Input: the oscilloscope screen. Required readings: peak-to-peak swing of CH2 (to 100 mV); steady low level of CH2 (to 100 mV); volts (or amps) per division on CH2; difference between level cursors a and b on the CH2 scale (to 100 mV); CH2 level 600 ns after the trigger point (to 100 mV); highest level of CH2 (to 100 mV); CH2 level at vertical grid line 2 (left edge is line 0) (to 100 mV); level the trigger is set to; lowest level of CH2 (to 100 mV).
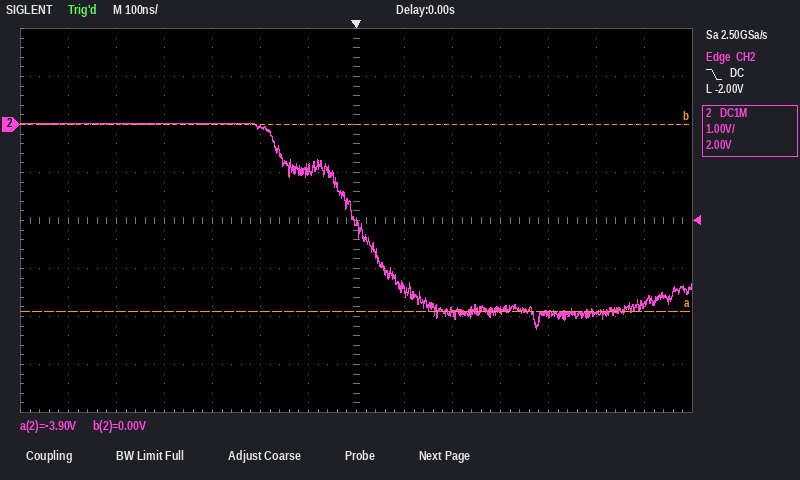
4.3 V
-3.9 V
1 V
3.9 V
-3.8 V
0.0 V
0.0 V
-2.00 V
-4.3 V
